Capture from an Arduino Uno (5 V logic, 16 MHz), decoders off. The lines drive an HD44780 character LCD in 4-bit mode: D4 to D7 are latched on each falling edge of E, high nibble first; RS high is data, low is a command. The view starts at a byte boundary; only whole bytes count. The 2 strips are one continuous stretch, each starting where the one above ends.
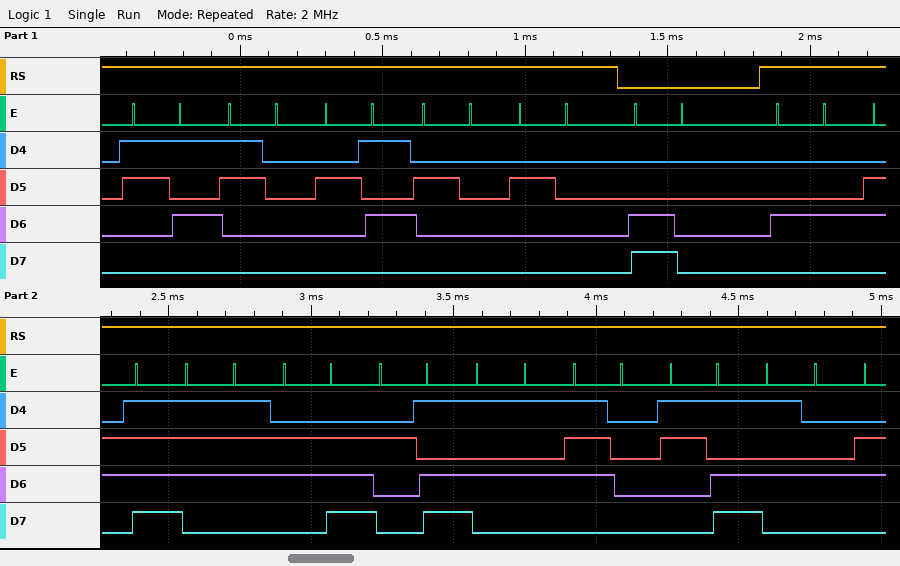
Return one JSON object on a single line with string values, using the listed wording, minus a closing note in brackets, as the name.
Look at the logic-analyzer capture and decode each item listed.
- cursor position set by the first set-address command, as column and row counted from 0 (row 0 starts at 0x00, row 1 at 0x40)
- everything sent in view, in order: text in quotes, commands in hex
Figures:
{"cursor position set by the first set-address command, as column and row counted from 0": "column 0, row 1", "everything sent in view, in order: text in quotes, commands in hex": "\"50%  \" 0xC0 \"Down-Up=T\""}
